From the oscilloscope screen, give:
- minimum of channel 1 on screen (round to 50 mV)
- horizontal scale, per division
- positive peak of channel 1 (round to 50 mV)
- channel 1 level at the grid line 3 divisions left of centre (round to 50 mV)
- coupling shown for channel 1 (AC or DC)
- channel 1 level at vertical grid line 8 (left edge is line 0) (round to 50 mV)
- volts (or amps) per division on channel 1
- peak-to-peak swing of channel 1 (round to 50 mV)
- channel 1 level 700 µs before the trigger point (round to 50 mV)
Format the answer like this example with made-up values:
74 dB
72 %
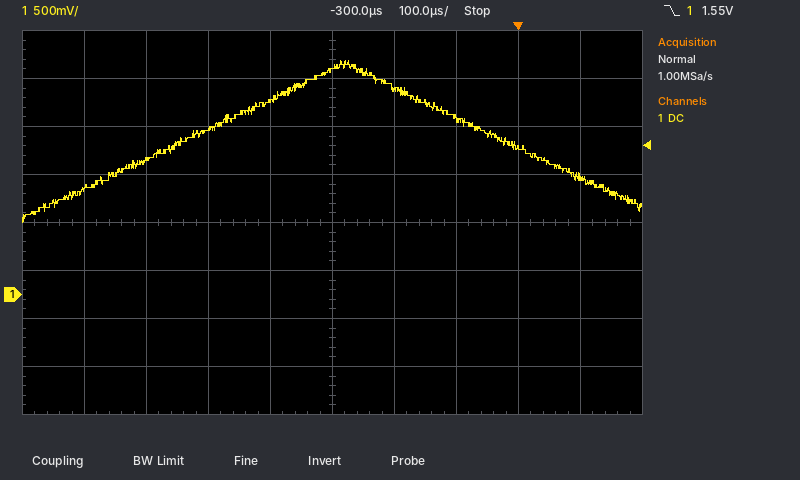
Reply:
750 mV
100 µs
2.45 V
1.40 V
DC
1.55 V
500 mV
1.70 V
1.10 V
